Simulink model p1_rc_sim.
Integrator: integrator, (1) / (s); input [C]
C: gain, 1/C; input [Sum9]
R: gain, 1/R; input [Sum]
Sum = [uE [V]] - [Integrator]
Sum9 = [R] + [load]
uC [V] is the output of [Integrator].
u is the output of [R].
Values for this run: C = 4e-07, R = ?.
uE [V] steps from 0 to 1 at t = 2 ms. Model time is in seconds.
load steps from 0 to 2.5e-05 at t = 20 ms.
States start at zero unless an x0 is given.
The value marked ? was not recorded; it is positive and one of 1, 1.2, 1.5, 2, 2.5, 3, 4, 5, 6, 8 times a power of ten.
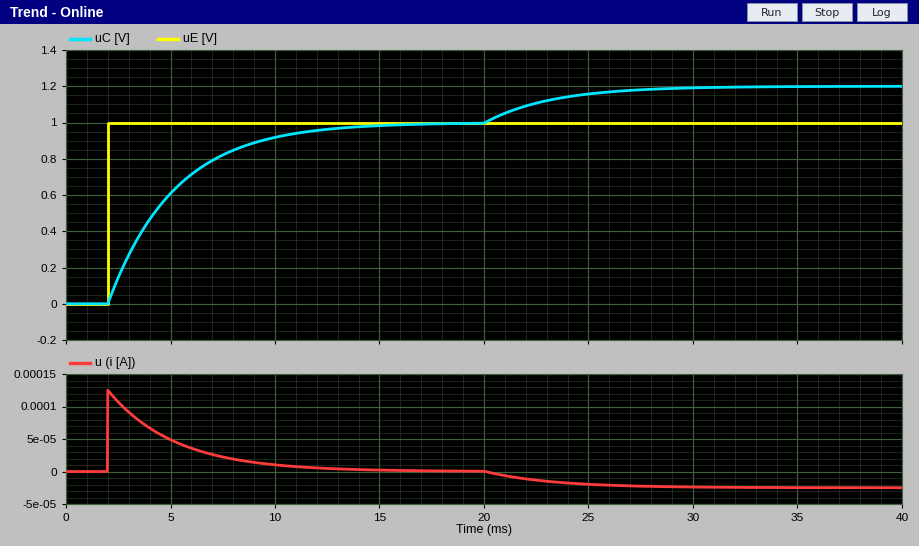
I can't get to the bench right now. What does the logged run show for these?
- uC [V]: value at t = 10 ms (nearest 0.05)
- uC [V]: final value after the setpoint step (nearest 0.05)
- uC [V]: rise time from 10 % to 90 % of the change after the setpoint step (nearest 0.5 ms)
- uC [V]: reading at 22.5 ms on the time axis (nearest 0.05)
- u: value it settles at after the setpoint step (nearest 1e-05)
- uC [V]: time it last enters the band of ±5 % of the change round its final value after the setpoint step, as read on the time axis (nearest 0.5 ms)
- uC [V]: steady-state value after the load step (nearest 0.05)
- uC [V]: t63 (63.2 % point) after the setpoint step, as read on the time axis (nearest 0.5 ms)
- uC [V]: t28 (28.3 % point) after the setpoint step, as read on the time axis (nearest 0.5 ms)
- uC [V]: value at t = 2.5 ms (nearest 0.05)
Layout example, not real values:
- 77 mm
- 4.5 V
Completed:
- 0.90
- 1.00
- 7.0 ms
- 1.10
- 0.00000
- 11.5 ms
- 1.20
- 5.0 ms
- 3.0 ms
- 0.15
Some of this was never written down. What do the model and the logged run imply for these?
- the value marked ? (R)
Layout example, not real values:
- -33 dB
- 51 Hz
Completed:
- 8000
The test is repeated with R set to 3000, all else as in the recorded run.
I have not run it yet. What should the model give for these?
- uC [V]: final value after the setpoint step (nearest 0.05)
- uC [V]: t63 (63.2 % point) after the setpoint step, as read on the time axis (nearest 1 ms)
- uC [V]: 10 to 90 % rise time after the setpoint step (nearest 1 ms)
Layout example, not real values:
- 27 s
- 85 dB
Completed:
- 1.00
- 3 ms
- 3 ms
